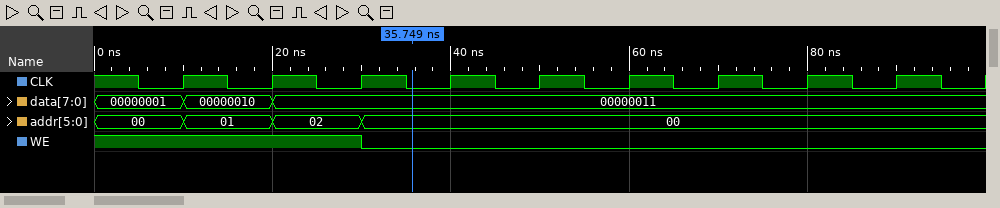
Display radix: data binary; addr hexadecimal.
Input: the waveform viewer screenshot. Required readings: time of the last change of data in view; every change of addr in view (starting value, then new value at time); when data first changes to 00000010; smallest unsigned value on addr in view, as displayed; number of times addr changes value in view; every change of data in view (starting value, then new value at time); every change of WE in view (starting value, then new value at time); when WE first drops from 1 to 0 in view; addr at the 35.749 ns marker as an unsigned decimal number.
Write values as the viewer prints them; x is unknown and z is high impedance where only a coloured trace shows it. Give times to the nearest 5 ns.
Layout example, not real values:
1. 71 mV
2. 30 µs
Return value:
1. 20 ns
2. 00, 01 at 10 ns, 02 at 20 ns, 00 at 30 ns
3. 10 ns
4. 00
5. 3
6. 00000001, 00000010 at 10 ns, 00000011 at 20 ns
7. 1, 0 at 30 ns
8. 30 ns
9. 0
